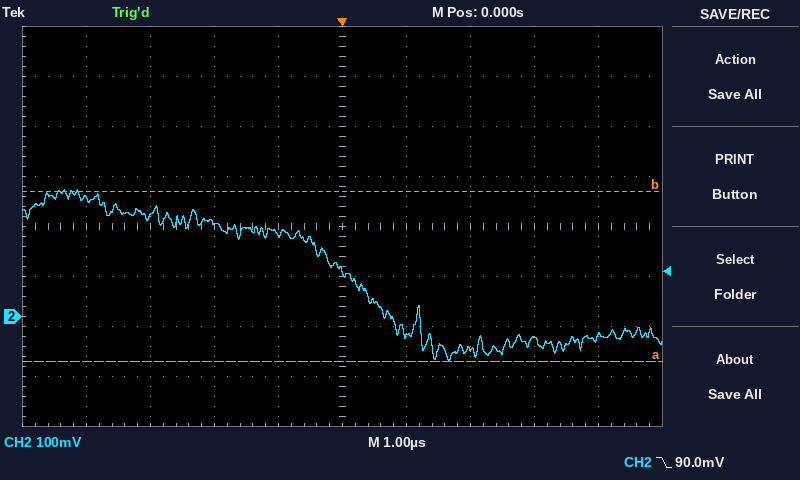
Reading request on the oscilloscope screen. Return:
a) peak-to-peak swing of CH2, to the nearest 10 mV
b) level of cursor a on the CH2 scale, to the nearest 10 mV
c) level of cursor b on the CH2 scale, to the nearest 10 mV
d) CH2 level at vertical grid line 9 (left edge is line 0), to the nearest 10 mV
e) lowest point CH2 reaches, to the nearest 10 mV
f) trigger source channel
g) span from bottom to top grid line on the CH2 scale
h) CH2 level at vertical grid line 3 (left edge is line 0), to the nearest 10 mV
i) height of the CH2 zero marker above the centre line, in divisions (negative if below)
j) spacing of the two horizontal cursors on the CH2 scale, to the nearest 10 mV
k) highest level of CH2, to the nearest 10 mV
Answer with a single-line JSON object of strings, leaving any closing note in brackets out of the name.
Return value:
{"peak-to-peak swing of CH2, to the nearest 10 mV": "340 mV", "level of cursor a on the CH2 scale, to the nearest 10 mV": "-90 mV", "level of cursor b on the CH2 scale, to the nearest 10 mV": "250 mV", "CH2 level at vertical grid line 9 (left edge is line 0), to the nearest 10 mV": "-40 mV", "lowest point CH2 reaches, to the nearest 10 mV": "-90 mV", "trigger source channel": "CH2", "span from bottom to top grid line on the CH2 scale": "800 mV", "CH2 level at vertical grid line 3 (left edge is line 0), to the nearest 10 mV": "190 mV", "height of the CH2 zero marker above the centre line, in divisions": "-1.8 div", "spacing of the two horizontal cursors on the CH2 scale, to the nearest 10 mV": "340 mV", "highest level of CH2, to the nearest 10 mV": "250 mV"}
